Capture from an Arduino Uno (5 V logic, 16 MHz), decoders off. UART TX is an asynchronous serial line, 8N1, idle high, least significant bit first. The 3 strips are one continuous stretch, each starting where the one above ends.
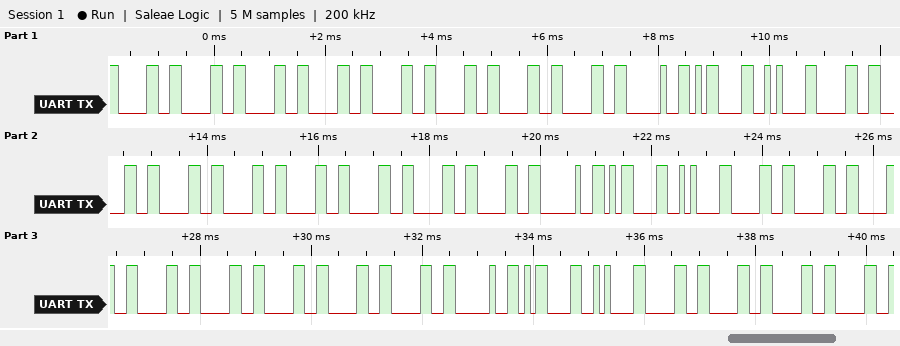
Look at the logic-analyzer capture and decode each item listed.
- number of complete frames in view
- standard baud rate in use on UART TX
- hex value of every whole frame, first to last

37
9600 baud
30 30 30 30 30 30 30 30 20 0D 0A 30 30 30 30 30 30 30 30 20 0D 0A 30 30 30 30 30 30 30 30 20 0D 0A 30 30 30 30
